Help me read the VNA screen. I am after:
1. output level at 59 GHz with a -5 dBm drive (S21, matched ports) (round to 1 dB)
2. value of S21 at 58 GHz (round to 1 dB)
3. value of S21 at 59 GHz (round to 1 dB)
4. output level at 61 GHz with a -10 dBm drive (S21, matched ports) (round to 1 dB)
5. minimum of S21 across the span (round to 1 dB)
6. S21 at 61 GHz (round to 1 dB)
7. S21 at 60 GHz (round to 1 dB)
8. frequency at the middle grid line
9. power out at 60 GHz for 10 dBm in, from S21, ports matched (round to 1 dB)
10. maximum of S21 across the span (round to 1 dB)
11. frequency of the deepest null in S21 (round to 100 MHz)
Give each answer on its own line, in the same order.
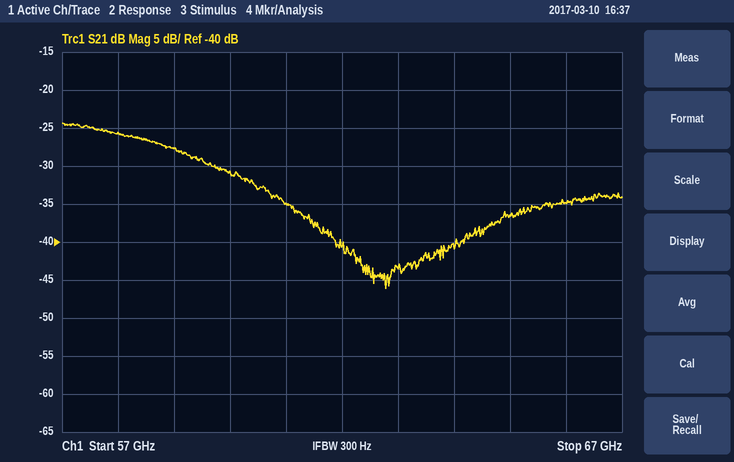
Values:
-33 dBm
-26 dB
-28 dB
-45 dBm
-46 dB
-35 dB
-31 dB
62 GHz
-21 dBm
-24 dB
62.8 GHz
